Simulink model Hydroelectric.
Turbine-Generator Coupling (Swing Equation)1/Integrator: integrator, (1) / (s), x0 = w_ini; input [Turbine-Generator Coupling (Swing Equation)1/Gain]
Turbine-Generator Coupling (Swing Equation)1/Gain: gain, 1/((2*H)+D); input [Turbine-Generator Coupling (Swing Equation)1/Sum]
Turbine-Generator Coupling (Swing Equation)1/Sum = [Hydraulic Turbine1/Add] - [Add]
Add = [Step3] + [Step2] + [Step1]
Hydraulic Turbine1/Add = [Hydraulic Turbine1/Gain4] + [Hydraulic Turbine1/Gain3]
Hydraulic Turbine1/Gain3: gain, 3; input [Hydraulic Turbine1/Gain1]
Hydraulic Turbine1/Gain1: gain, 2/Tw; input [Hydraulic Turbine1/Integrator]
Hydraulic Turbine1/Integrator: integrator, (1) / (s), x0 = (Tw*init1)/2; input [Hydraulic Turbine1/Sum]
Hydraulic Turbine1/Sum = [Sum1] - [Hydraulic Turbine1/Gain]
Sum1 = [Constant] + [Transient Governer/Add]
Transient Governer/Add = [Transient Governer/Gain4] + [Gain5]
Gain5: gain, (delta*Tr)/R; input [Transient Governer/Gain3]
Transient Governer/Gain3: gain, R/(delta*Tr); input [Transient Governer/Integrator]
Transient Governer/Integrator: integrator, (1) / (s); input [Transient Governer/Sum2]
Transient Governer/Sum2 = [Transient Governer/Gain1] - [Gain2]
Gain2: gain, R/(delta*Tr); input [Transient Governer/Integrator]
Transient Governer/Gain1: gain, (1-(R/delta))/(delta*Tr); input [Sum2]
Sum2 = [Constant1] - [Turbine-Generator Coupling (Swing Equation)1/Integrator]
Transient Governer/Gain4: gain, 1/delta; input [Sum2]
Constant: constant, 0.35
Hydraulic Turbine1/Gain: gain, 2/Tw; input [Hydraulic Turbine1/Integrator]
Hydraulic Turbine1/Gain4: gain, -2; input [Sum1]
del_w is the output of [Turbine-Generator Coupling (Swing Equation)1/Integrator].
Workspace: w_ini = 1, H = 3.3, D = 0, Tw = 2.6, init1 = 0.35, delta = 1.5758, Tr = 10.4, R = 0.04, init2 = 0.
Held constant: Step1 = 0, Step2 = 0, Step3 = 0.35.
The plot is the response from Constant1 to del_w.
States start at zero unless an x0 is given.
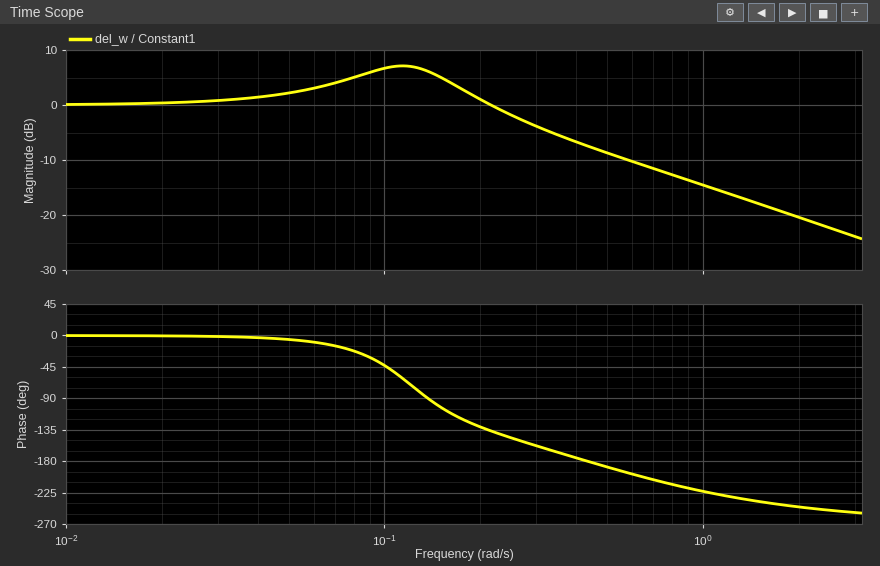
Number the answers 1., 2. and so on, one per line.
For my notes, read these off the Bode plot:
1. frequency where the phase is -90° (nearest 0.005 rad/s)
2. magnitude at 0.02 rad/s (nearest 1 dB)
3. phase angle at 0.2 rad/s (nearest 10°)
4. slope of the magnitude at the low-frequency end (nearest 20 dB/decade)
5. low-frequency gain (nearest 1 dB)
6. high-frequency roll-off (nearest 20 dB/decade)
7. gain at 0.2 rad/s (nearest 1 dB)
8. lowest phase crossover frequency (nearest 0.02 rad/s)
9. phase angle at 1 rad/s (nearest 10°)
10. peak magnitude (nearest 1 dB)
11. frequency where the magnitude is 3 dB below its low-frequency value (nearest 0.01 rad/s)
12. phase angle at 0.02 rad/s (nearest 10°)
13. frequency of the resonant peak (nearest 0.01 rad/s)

1. 0.135 rad/s
2. 0 dB
3. -130°
4. 0 dB/decade
5. 0 dB
6. -20 dB/decade
7. 1 dB
8. 0.44 rad/s
9. -220°
10. 7 dB
11. 0.27 rad/s
12. 0°
13. 0.11 rad/s
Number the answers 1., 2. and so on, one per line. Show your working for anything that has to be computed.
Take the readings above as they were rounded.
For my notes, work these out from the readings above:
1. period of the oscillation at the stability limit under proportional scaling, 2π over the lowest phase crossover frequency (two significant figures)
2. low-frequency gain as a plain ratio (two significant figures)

1. 2π / 0.44 = 14 s
2. 10^(0 / 20) = 1.0
